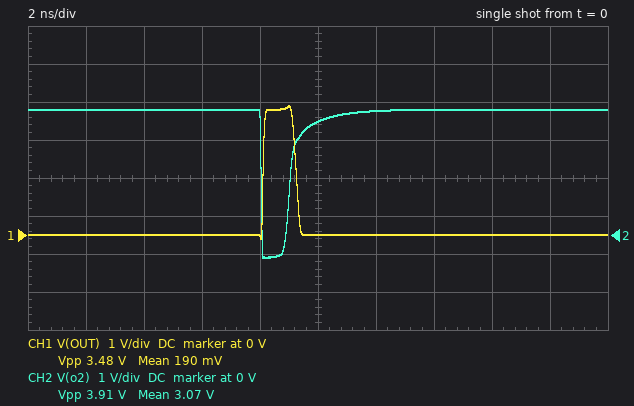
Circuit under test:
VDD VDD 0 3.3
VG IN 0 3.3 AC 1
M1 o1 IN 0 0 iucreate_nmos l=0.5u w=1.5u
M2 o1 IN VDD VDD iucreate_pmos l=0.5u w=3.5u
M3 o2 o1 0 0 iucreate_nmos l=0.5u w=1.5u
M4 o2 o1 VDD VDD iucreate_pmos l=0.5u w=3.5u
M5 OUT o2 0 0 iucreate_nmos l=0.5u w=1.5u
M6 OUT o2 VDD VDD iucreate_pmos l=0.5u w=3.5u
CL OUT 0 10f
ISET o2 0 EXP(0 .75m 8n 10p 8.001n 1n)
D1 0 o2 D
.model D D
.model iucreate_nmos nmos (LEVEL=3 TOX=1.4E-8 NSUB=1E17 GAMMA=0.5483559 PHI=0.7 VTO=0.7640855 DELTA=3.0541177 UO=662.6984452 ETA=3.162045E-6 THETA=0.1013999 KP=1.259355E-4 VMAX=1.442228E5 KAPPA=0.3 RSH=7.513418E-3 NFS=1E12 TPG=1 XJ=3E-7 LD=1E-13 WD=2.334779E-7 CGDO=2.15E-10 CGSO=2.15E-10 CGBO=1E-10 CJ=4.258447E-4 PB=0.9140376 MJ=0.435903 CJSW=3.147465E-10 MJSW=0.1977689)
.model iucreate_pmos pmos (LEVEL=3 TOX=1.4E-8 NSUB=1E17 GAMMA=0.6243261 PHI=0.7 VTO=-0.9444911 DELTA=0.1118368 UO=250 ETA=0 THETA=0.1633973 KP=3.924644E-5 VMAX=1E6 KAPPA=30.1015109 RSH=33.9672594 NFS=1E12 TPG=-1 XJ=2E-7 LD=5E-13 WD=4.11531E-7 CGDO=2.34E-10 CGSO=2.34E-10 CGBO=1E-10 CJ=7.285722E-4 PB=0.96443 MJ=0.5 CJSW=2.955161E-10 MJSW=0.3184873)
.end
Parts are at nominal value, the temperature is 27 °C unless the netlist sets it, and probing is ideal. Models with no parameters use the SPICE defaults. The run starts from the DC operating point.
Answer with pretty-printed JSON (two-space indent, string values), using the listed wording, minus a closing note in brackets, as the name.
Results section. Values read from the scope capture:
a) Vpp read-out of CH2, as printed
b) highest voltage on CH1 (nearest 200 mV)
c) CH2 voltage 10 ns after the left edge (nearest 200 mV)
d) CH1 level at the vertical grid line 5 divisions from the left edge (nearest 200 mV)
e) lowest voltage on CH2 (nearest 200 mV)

{
  "Vpp read-out of CH2, as printed": "3.91 V",
  "highest voltage on CH1": "3.4 V",
  "CH2 voltage 10 ns after the left edge": "3.0 V",
  "CH1 level at the vertical grid line 5 divisions from the left edge": "0 V",
  "lowest voltage on CH2": "-600 mV"
}
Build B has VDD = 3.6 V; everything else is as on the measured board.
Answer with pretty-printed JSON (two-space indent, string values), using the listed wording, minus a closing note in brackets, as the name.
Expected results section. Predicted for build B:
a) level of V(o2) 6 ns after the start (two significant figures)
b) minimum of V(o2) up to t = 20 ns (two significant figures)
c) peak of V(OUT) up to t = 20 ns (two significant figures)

{
  "level of V(o2) 6 ns after the start": "3.6 V",
  "minimum of V(o2) up to t = 20 ns": "-590 mV",
  "peak of V(OUT) up to t = 20 ns": "3.7 V"
}
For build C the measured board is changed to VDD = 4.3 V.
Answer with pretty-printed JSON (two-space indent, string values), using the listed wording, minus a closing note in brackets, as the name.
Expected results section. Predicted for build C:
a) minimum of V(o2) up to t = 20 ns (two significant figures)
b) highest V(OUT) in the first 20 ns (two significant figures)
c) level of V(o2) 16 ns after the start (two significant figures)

{
  "minimum of V(o2) up to t = 20 ns": "1.6 V",
  "highest V(OUT) in the first 20 ns": "2.6 V",
  "level of V(o2) 16 ns after the start": "4.3 V"
}
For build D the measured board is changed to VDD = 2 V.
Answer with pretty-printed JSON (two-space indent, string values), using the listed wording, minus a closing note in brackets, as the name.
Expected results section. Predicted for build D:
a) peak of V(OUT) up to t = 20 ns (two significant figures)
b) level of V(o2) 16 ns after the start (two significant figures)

{
  "peak of V(OUT) up to t = 20 ns": "2.1 V",
  "level of V(o2) 16 ns after the start": "2.0 V"
}
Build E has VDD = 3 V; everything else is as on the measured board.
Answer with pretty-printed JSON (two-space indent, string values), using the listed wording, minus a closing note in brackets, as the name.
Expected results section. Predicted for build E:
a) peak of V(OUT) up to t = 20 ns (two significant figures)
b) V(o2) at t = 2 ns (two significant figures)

{
  "peak of V(OUT) up to t = 20 ns": "3.1 V",
  "V(o2) at t = 2 ns": "3.0 V"
}
